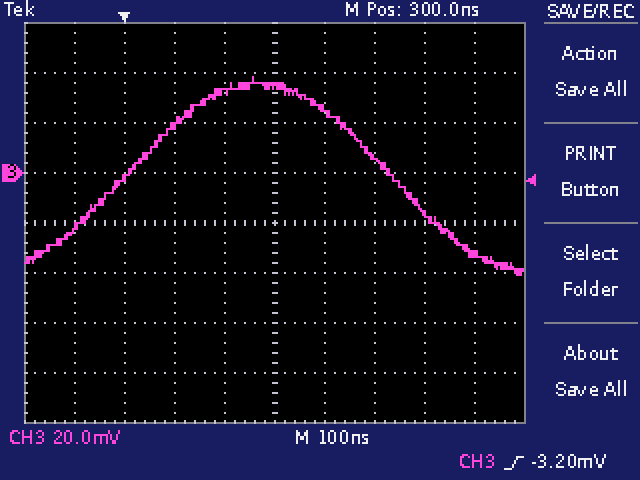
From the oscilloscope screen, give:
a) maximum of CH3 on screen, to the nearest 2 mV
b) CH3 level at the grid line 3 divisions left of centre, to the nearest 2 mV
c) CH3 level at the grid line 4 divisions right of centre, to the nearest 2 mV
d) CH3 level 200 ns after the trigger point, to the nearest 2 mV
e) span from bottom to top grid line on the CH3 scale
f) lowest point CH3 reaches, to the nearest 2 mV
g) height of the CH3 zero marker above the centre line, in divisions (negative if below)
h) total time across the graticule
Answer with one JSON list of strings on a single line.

["38 mV", "-2 mV", "-32 mV", "32 mV", "160 mV", "-40 mV", "+1.0 div", "1 µs"]
